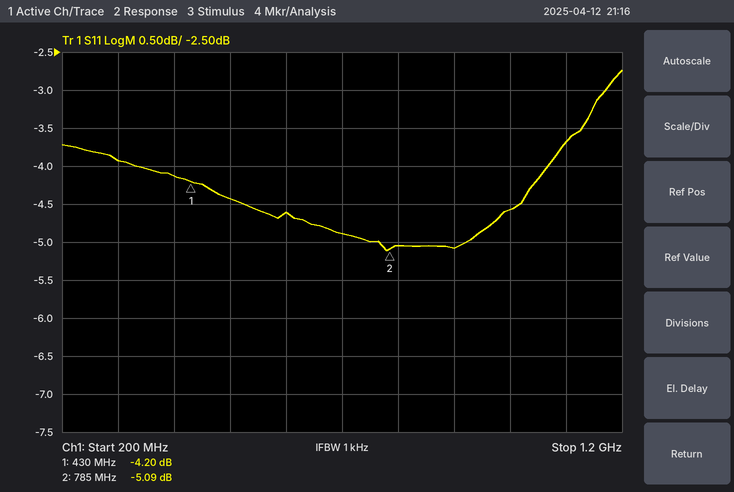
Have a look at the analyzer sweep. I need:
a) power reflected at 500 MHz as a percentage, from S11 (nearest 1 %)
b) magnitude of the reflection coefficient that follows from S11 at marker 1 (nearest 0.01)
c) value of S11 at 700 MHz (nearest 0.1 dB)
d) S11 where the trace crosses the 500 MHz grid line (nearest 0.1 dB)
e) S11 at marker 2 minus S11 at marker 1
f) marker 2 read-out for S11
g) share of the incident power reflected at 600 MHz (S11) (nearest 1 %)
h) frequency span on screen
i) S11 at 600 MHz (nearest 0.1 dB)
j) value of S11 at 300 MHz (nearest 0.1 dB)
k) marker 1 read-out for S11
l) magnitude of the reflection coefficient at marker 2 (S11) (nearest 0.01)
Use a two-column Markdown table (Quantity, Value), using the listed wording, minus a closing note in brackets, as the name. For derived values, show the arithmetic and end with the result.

| Quantity | Value |
|---|---|
| power reflected at 500 MHz as a percentage, from S11 | 10^(-4.4/10) ≈ 36 % |
| magnitude of the reflection coefficient that follows from S11 at marker 1 | 10^(-4.2/20) ≈ 0.62 |
| value of S11 at 700 MHz | -4.9 dB |
| S11 where the trace crosses the 500 MHz grid line | -4.4 dB |
| S11 at marker 2 minus S11 at marker 1 | -5.09 − (-4.2) = -0.89 dB |
| marker 2 read-out for S11 | -5.09 dB |
| share of the incident power reflected at 600 MHz (S11) | 10^(-4.6/10) ≈ 35 % |
| frequency span on screen | 1 GHz |
| S11 at 600 MHz | -4.6 dB |
| value of S11 at 300 MHz | -3.9 dB |
| marker 1 read-out for S11 | -4.20 dB |
| magnitude of the reflection coefficient at marker 2 (S11) | 10^(-5.09/20) ≈ 0.56 |
